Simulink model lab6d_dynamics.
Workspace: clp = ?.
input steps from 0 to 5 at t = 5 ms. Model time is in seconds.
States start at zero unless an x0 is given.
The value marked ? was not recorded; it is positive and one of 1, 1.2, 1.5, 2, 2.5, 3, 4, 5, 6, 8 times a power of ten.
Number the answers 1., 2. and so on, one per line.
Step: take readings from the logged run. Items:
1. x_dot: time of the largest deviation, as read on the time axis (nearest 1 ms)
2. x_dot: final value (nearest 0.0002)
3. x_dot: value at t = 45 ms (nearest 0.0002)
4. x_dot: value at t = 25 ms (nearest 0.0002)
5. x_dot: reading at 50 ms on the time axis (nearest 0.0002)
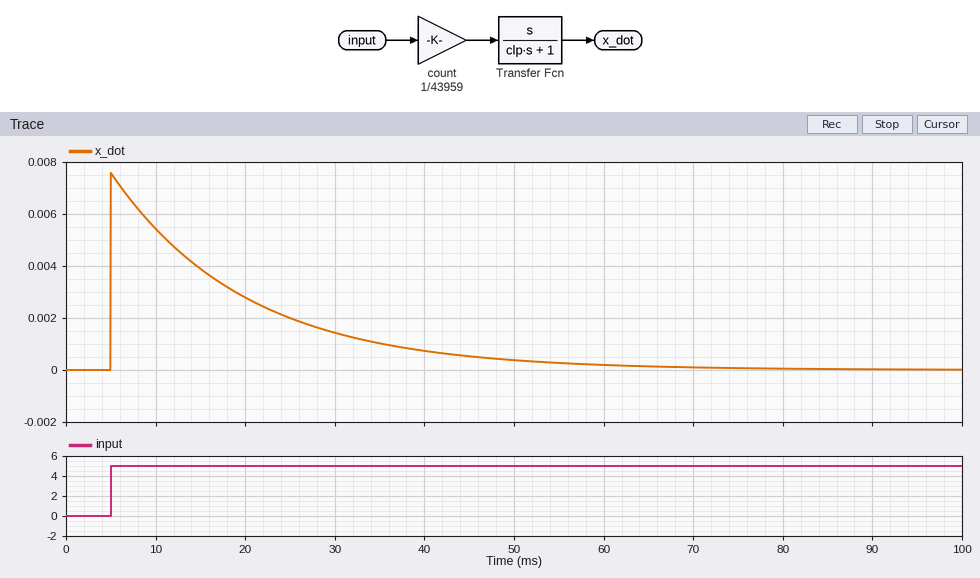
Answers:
1. 5 ms
2. 0.0000
3. 0.0006
4. 0.0020
5. 0.0004
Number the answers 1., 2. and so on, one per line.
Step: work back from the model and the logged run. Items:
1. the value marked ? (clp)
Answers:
1. 0.015
